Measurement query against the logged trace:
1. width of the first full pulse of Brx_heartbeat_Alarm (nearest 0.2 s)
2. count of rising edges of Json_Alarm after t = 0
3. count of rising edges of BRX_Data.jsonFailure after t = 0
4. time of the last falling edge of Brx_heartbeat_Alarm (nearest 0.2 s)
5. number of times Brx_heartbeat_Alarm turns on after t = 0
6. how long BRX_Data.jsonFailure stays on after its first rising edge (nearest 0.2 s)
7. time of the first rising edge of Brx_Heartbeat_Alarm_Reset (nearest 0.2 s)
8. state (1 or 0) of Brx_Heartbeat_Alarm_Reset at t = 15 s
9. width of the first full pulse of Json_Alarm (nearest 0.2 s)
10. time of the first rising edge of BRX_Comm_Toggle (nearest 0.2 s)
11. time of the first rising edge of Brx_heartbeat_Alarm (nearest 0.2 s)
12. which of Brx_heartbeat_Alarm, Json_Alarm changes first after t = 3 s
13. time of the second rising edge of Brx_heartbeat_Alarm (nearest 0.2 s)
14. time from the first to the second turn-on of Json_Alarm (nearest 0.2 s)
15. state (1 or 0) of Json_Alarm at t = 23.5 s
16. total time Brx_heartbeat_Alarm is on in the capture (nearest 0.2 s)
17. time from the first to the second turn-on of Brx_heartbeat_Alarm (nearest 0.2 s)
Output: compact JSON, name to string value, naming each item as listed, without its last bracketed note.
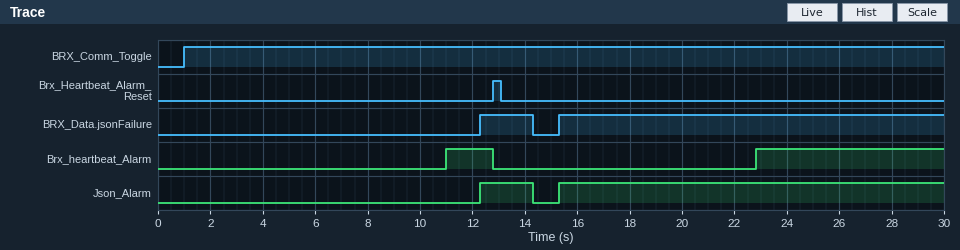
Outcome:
{"width of the first full pulse of Brx_heartbeat_Alarm": "1.8 s", "count of rising edges of Json_Alarm after t = 0": "2", "count of rising edges of BRX_Data.jsonFailure after t = 0": "2", "time of the last falling edge of Brx_heartbeat_Alarm": "12.8 s", "number of times Brx_heartbeat_Alarm turns on after t = 0": "2", "how long BRX_Data.jsonFailure stays on after its first rising edge": "2.0 s", "time of the first rising edge of Brx_Heartbeat_Alarm_Reset": "12.8 s", "state (1 or 0) of Brx_Heartbeat_Alarm_Reset at t = 15 s": "0", "width of the first full pulse of Json_Alarm": "2.0 s", "time of the first rising edge of BRX_Comm_Toggle": "1.0 s", "time of the first rising edge of Brx_heartbeat_Alarm": "11.0 s", "which of Brx_heartbeat_Alarm, Json_Alarm changes first after t = 3 s": "Brx_heartbeat_Alarm", "time of the second rising edge of Brx_heartbeat_Alarm": "22.8 s", "time from the first to the second turn-on of Json_Alarm": "3.0 s", "state (1 or 0) of Json_Alarm at t = 23.5 s": "1", "total time Brx_heartbeat_Alarm is on in the capture": "9.0 s", "time from the first to the second turn-on of Brx_heartbeat_Alarm": "11.8 s"}
